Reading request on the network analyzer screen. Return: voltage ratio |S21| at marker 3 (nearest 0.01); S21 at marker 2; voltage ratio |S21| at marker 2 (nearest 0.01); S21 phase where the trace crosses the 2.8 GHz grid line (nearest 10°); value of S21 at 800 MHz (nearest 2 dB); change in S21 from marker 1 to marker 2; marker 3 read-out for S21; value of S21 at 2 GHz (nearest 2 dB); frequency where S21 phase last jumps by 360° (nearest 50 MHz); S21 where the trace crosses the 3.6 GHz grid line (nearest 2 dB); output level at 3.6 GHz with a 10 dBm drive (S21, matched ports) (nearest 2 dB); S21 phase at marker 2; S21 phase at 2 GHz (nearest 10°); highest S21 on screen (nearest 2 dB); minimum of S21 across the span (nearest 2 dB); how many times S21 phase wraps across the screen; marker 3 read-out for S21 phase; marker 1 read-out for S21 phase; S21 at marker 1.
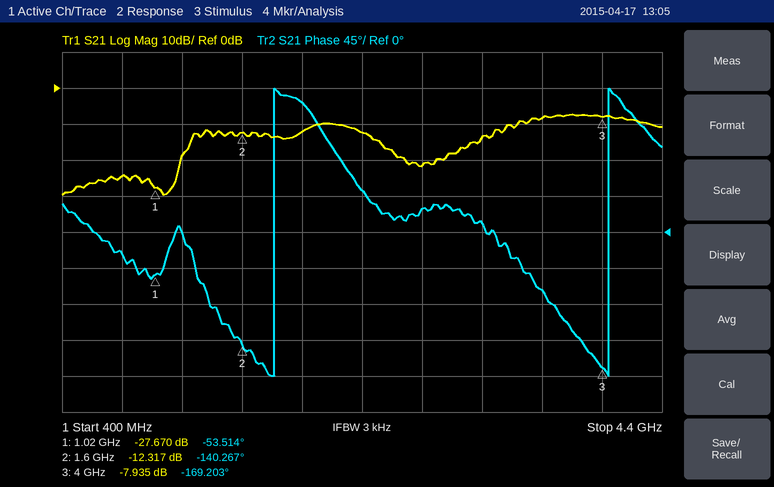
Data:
0.40
-12.317 dB
0.24
30°
-24 dB
15.353 dB
-7.935 dB
-12 dB
4.05 GHz
-8 dB
2 dBm
-140.267°
160°
-8 dB
-30 dB
2
-169.203°
-53.514°
-27.670 dB
